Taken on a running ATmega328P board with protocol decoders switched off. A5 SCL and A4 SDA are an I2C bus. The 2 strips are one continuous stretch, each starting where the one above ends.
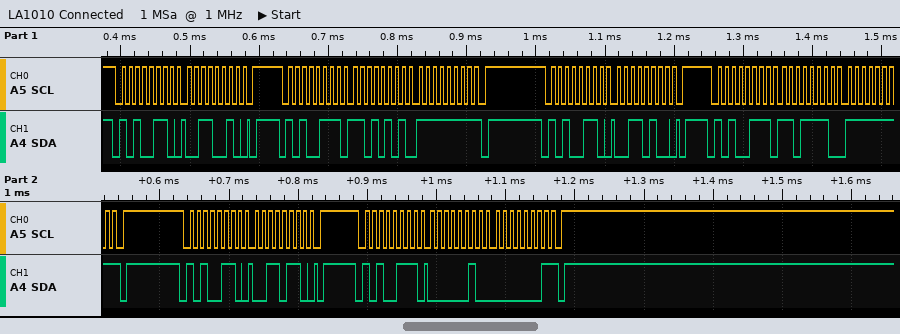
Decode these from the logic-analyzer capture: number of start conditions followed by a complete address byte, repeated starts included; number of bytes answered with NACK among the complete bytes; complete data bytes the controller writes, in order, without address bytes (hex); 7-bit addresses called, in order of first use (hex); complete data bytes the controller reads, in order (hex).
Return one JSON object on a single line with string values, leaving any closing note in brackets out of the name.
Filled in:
{"number of start conditions followed by a complete address byte, repeated starts included": "6", "number of bytes answered with NACK among the complete bytes": "3", "complete data bytes the controller writes, in order, without address bytes": "32 34 36", "7-bit addresses called, in order of first use": "0x53", "complete data bytes the controller reads, in order": "D5 FF DE FF 02 01"}
